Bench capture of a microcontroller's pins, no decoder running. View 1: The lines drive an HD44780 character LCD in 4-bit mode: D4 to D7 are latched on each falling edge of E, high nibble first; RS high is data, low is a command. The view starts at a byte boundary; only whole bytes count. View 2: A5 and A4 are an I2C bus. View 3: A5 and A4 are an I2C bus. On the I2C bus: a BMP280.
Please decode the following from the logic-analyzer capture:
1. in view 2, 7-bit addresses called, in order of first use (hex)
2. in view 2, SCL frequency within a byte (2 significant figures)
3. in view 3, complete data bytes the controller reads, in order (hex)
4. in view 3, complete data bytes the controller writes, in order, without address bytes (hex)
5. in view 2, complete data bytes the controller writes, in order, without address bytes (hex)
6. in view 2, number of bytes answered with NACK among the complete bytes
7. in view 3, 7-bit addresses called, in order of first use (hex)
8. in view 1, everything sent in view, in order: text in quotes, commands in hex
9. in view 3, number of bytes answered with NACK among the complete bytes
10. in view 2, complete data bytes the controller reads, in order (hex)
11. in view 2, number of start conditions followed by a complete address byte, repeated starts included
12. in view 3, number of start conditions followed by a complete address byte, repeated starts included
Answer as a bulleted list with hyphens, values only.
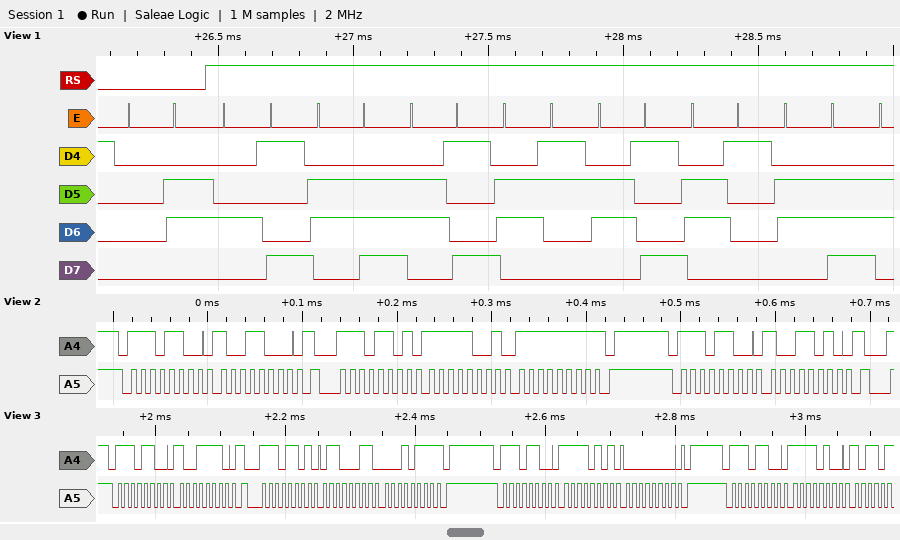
- 0x76
- 100 kHz
- 63 17
- 9E F5 00 F4
- 98 9A
- 1
- 0x76
- 0x06 "Inician"
- 1
- F9 FF
- 3
- 4
